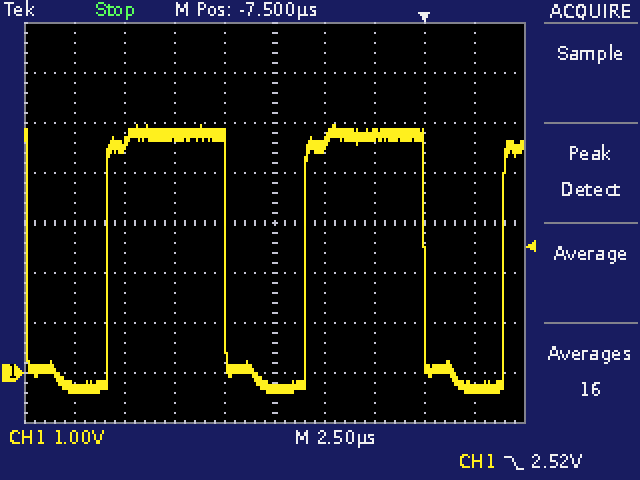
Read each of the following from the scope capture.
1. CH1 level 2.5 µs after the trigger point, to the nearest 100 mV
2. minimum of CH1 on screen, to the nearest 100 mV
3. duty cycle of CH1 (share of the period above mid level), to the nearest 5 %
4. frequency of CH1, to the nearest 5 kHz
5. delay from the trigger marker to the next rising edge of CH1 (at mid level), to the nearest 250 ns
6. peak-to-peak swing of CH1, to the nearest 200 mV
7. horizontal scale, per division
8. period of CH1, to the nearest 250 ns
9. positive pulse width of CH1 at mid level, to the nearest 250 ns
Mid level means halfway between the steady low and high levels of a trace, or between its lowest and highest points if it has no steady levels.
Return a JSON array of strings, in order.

["-300 mV", "-400 mV", "60 %", "100 kHz", "4.00 µs", "5.4 V", "2.5 µs", "10.00 µs", "6.00 µs"]
